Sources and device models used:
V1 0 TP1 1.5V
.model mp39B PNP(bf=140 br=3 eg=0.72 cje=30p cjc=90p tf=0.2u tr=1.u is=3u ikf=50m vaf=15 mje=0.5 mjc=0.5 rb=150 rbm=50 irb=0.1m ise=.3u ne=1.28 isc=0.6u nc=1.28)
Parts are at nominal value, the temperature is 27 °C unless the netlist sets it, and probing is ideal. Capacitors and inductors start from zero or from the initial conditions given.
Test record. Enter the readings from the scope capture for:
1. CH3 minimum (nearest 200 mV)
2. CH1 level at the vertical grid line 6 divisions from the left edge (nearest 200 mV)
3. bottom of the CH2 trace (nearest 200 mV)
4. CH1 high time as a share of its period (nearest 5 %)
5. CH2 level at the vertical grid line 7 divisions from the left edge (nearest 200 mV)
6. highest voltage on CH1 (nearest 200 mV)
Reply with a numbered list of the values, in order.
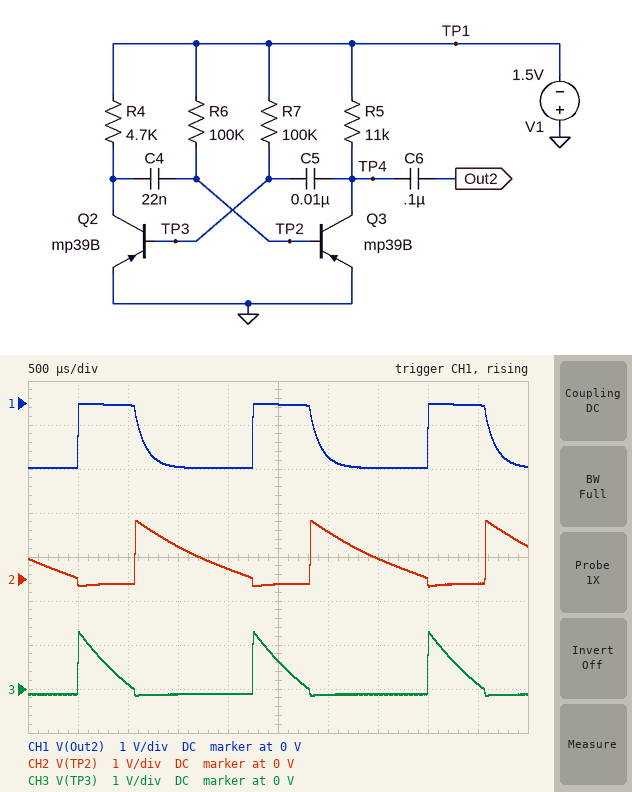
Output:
1. -200 mV
2. -1.2 V
3. -200 mV
4. 35 %
5. 400 mV
6. 0 V
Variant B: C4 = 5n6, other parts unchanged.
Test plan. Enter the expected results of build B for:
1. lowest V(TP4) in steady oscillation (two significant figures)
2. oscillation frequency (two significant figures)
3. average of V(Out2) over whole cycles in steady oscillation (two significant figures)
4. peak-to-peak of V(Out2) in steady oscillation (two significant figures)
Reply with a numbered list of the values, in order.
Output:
1. -1.4 V
2. 1.2 kHz
3. -420 mV
4. 1.4 V
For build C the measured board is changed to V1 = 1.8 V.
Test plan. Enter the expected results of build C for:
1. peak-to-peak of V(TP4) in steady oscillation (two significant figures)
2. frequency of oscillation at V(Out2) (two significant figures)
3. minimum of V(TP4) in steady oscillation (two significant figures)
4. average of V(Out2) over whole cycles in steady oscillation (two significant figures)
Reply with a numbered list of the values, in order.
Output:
1. 1.8 V
2. 550 Hz
3. -1.8 V
4. -1.1 V
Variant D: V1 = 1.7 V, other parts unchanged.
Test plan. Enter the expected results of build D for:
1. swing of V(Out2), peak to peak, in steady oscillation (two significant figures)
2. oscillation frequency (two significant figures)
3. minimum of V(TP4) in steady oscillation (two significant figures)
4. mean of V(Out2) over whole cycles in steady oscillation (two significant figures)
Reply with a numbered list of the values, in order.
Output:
1. 1.7 V
2. 550 Hz
3. -1.7 V
4. -1.1 V
